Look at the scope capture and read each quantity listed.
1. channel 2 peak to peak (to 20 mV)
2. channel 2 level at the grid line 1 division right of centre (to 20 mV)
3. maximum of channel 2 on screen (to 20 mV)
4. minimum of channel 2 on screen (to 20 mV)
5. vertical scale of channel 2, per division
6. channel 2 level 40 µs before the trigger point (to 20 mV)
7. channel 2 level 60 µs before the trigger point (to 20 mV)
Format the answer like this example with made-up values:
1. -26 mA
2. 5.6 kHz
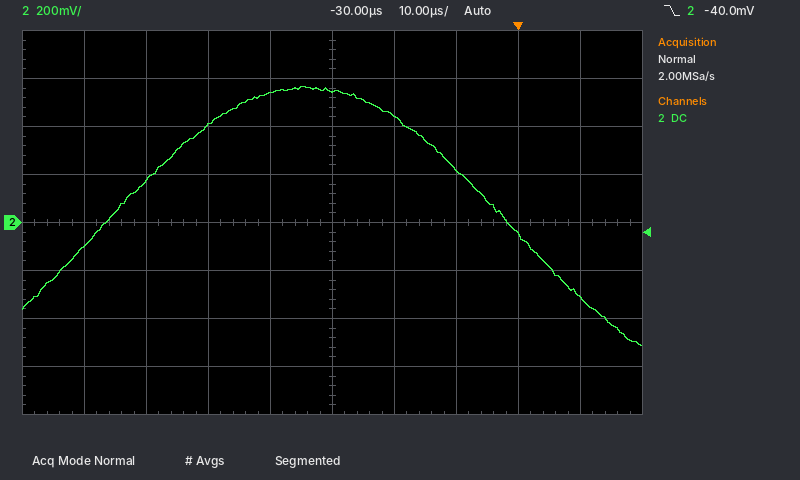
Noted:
1. 1.08 V
2. 440 mV
3. 560 mV
4. -520 mV
5. 200 mV
6. 540 mV
7. 180 mV
